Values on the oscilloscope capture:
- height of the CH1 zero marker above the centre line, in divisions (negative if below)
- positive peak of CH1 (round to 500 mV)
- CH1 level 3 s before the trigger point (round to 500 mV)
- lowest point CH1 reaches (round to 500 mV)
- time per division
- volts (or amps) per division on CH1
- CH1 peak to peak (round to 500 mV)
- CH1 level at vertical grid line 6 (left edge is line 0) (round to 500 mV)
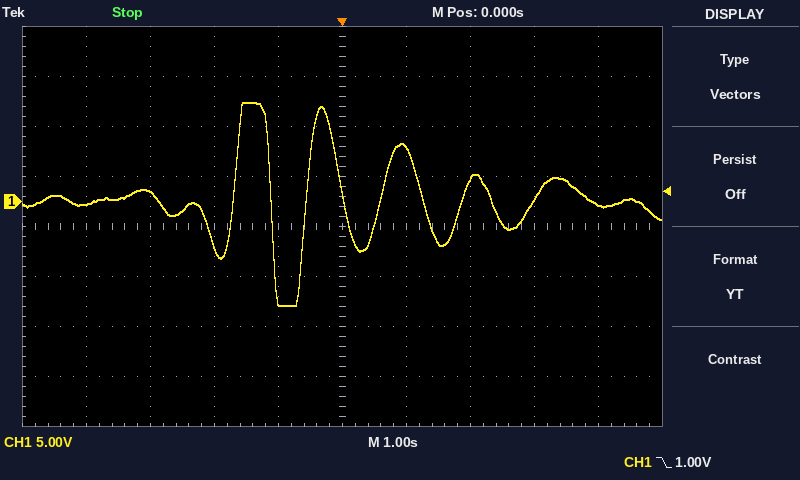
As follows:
+0.5 div
10.0 V
1.0 V
-10.5 V
1 s
5 V
20.5 V
5.5 V
